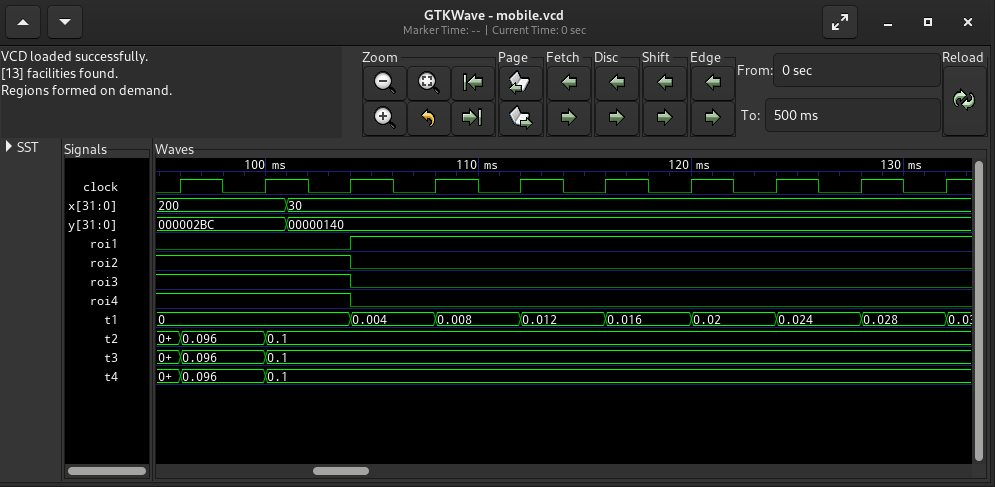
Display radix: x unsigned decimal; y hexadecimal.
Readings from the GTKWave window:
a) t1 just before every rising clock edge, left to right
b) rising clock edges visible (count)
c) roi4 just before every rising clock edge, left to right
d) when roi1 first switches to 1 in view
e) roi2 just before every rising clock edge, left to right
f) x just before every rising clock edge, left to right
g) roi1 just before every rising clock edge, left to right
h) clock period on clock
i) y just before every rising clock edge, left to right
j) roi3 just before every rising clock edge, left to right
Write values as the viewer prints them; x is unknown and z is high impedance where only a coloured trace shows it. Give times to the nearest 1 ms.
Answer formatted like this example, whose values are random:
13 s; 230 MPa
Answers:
0, 0, 0, 0.004, 0.008, 0.012, 0.016, 0.02, 0.024, 0.028; 10; 1 1 1 0 0 0 0 0 0 0; 104 ms; 1 1 1 0 0 0 0 0 0 0; 200, 200, 30, 30, 30, 30, 30, 30, 30, 30; 0 0 0 1 1 1 1 1 1 1; 4 ms; 000002BC, 000002BC, 00000140, 00000140, 00000140, 00000140, 00000140, 00000140, 00000140, 00000140; 1 1 1 0 0 0 0 0 0 0
